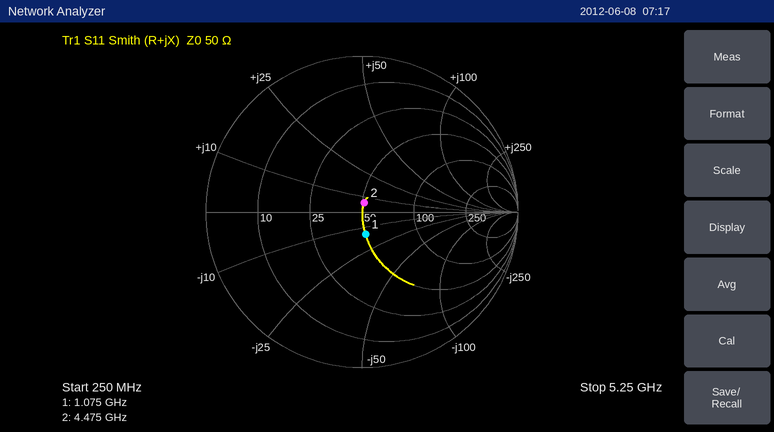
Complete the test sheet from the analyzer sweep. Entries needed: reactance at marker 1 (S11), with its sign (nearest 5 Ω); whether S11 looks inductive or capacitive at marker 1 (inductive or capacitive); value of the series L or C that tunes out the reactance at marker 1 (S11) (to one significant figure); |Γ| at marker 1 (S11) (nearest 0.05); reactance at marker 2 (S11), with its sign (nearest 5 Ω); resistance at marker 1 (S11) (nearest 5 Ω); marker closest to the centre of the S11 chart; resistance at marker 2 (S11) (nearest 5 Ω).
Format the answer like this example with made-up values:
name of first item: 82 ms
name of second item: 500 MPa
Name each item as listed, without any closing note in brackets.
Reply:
reactance at marker 1 (S11), with its sign: -15 Ω
whether S11 looks inductive or capacitive at marker 1: capacitive
value of the series L or C that tunes out the reactance at marker 1 (S11): 2 nH
|Γ| at marker 1 (S11): 0.15
reactance at marker 2 (S11), with its sign: +5 Ω
resistance at marker 1 (S11): 50 Ω
marker closest to the centre of the S11 chart: marker 2
resistance at marker 2 (S11): 50 Ω
